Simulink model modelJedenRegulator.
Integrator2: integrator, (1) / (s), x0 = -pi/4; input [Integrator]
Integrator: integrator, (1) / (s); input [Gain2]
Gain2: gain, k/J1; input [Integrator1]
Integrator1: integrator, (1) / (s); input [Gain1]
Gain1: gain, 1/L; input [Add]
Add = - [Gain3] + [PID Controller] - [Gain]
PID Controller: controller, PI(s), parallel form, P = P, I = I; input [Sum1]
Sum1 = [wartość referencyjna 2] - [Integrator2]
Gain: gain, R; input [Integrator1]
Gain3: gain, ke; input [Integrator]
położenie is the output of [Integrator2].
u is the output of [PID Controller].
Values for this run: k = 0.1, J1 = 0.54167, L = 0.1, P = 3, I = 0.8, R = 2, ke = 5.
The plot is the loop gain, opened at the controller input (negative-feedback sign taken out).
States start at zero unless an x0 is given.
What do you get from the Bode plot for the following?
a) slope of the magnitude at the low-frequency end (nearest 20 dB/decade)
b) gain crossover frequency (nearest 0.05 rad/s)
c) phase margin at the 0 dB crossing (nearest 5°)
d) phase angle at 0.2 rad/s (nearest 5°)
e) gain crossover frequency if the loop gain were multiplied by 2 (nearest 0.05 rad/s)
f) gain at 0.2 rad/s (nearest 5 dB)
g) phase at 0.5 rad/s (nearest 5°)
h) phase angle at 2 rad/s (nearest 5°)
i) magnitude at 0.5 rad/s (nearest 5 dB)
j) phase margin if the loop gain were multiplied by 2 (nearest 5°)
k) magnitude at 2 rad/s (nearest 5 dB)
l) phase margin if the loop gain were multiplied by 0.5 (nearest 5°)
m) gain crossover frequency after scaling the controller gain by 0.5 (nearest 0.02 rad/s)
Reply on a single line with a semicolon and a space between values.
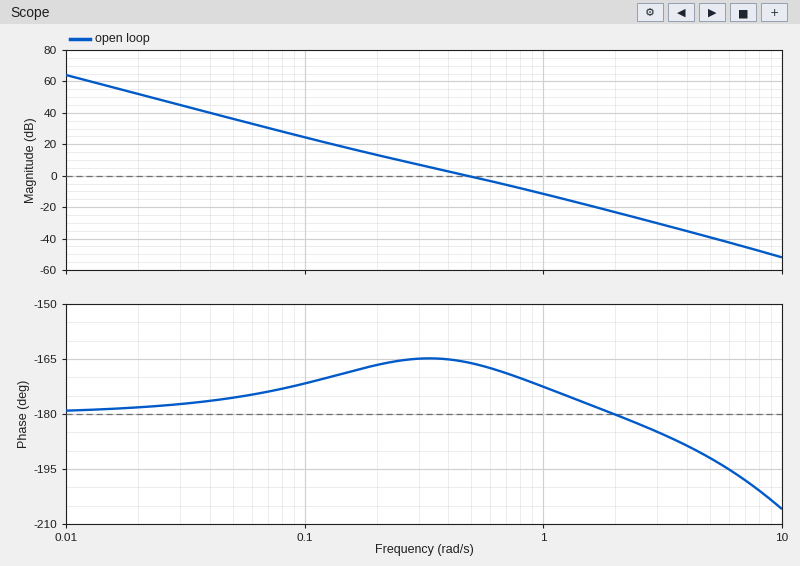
-40 dB/decade; 0.50 rad/s; 15°; -165°; 0.70 rad/s; 15 dB; -165°; -180°; 0 dB; 10°; -25 dB; 15°; 0.32 rad/s
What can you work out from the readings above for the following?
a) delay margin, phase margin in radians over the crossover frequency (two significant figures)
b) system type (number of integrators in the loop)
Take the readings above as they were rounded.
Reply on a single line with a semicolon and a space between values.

0.52 s; 2
